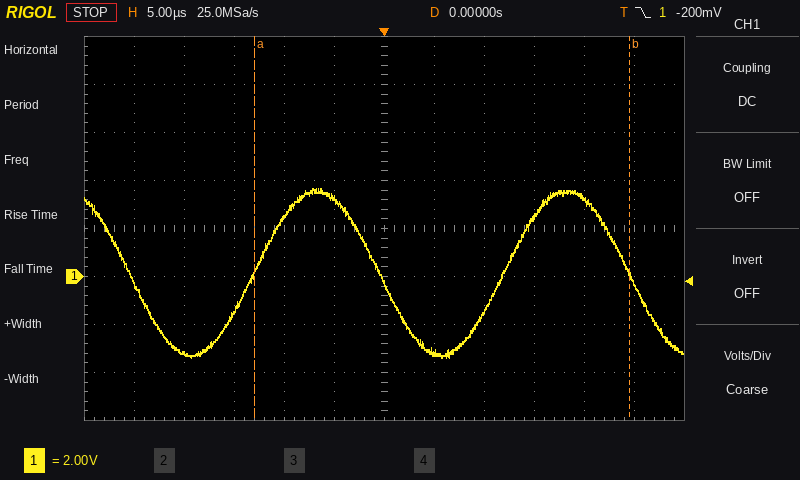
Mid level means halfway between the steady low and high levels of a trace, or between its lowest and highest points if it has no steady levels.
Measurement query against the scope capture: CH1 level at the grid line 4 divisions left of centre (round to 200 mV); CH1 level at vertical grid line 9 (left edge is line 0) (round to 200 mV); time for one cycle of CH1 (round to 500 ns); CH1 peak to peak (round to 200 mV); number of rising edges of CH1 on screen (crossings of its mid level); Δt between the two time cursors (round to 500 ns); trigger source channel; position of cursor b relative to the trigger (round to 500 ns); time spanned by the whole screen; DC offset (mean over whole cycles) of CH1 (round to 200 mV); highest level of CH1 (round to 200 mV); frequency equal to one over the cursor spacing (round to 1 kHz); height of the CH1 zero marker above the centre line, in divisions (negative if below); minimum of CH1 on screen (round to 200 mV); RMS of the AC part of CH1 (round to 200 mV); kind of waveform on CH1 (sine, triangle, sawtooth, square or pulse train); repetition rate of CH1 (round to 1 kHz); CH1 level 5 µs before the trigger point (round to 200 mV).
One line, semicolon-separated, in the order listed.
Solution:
-3.2 V; 2.4 V; 25.0 µs; 7.0 V; 2; 37.5 µs; CH1; +24.5 µs; 60 µs; 200 mV; 3.6 V; 27 kHz; -1.0 div; -3.4 V; 2.4 V; sine; 40 kHz; 3.2 V
